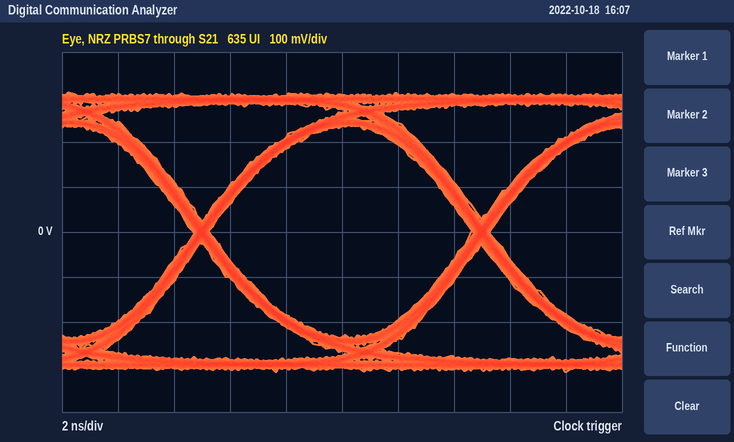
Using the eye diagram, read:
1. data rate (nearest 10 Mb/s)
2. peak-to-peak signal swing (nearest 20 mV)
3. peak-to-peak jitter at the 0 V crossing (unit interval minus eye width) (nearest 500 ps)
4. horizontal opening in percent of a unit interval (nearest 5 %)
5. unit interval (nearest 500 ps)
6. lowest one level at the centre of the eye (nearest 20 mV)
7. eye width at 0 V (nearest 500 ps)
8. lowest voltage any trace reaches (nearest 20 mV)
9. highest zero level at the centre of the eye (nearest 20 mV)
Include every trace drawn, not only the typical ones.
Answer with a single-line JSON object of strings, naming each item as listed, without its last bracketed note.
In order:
{"data rate": "100 Mb/s", "peak-to-peak signal swing": "620 mV", "peak-to-peak jitter at the 0 V crossing (unit interval minus eye width)": "500 ps", "horizontal opening in percent of a unit interval": "95 %", "unit interval": "10.0 ns", "lowest one level at the centre of the eye": "240 mV", "eye width at 0 V": "9.5 ns", "lowest voltage any trace reaches": "-320 mV", "highest zero level at the centre of the eye": "-240 mV"}
